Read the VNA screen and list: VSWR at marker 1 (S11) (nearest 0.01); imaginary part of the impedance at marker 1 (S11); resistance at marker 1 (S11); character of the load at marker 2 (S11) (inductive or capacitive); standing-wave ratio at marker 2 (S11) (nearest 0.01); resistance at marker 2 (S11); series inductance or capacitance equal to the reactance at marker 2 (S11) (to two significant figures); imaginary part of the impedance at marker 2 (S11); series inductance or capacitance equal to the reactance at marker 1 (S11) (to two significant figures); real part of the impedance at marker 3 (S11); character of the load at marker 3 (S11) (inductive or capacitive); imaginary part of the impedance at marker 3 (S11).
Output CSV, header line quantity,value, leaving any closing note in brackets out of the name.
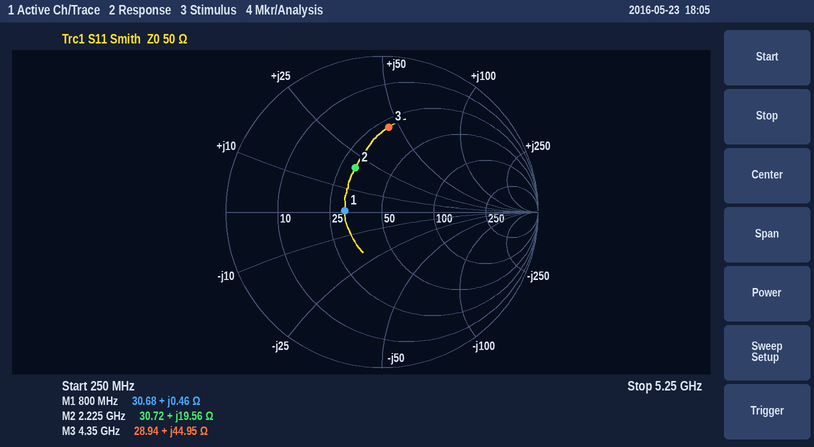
quantity,value
VSWR at marker 1 (S11),1.63
imaginary part of the impedance at marker 1,+0.46 Ω
resistance at marker 1,30.68 Ω
character of the load at marker 2 (S11),inductive
standing-wave ratio at marker 2 (S11),1.99
resistance at marker 2,30.72 Ω
series inductance or capacitance equal to the reactance at marker 2 (S11),1.4 nH
imaginary part of the impedance at marker 2,+19.56 Ω
series inductance or capacitance equal to the reactance at marker 1 (S11),92 pH
real part of the impedance at marker 3,28.94 Ω
character of the load at marker 3 (S11),inductive
imaginary part of the impedance at marker 3,+44.95 Ω
